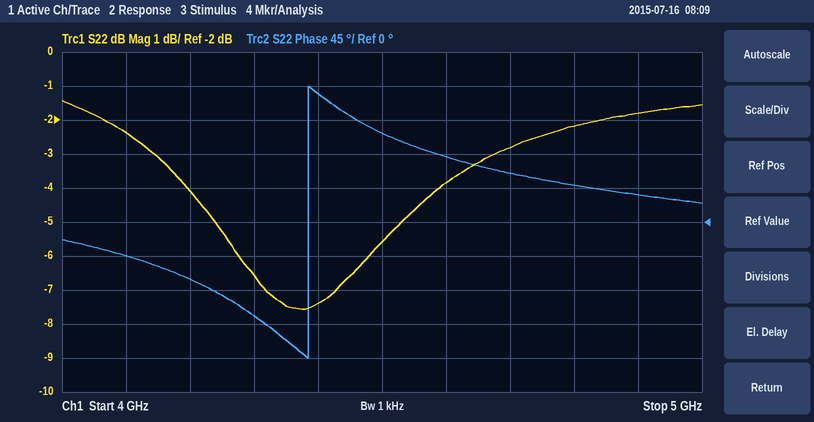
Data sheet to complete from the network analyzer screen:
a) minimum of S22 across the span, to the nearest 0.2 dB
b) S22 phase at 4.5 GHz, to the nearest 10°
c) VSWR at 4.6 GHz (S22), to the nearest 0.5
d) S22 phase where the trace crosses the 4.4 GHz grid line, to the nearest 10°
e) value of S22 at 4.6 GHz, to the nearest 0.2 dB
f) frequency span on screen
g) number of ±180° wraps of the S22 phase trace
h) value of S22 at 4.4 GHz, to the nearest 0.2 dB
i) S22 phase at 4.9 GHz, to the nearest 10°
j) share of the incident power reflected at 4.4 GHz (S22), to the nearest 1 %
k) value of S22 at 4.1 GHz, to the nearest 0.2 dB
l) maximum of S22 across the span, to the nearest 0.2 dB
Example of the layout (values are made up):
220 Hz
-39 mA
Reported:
-7.6 dB
120°
4.5
170°
-3.8 dB
1 GHz
1
-7.4 dB
40°
18 %
-2.4 dB
-1.4 dB
